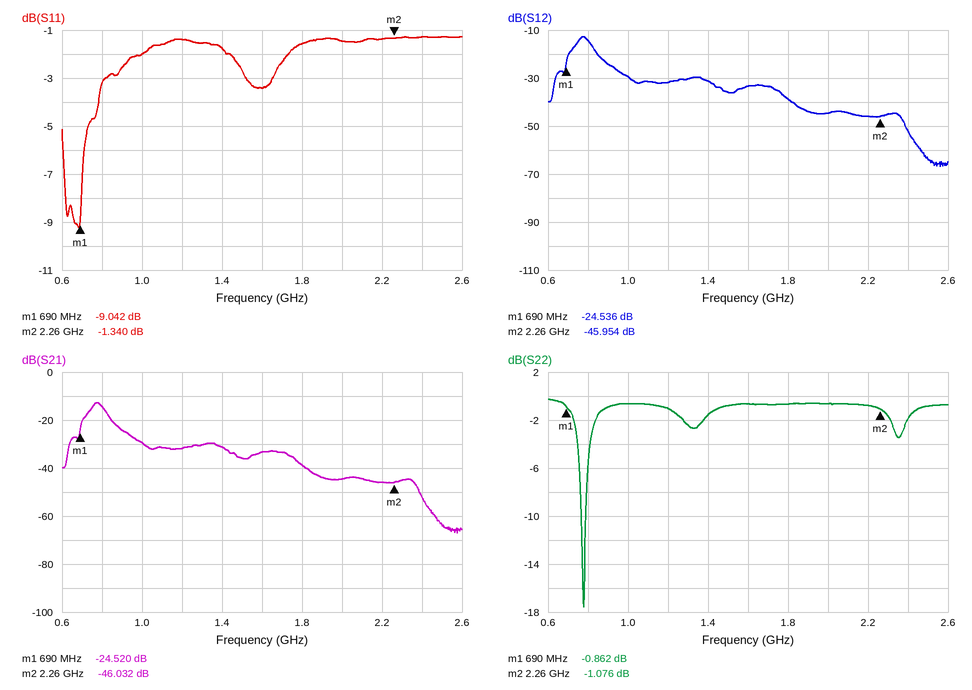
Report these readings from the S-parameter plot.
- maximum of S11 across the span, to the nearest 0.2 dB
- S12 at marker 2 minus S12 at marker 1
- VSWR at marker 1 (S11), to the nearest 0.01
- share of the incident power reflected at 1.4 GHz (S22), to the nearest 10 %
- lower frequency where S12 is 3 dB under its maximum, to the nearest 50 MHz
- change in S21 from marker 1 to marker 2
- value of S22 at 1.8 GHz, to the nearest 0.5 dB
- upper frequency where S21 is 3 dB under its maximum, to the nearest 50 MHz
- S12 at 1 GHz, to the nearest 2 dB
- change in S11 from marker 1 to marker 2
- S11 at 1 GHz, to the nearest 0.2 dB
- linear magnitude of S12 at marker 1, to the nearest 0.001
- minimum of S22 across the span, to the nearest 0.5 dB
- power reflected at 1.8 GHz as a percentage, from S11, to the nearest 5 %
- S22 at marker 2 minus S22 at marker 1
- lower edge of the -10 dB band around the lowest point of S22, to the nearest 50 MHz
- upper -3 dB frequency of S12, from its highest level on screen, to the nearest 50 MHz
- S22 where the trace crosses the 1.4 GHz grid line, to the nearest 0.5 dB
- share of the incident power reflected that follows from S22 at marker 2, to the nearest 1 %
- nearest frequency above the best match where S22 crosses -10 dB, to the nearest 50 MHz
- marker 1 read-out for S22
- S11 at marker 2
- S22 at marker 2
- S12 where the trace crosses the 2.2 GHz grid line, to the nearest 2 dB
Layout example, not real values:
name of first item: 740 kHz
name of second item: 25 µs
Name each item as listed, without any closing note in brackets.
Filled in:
maximum of S11 across the span, to the nearest 0.2 dB: -1.2 dB
S12 at marker 2 minus S12 at marker 1: -21.418 dB
VSWR at marker 1 (S11), to the nearest 0.01: 2.09
share of the incident power reflected at 1.4 GHz (S22), to the nearest 10 %: 70 %
lower frequency where S12 is 3 dB under its maximum, to the nearest 50 MHz: 750 MHz
change in S21 from marker 1 to marker 2: -21.512 dB
value of S22 at 1.8 GHz, to the nearest 0.5 dB: -0.5 dB
upper frequency where S21 is 3 dB under its maximum, to the nearest 50 MHz: 800 MHz
S12 at 1 GHz, to the nearest 2 dB: -30 dB
change in S11 from marker 1 to marker 2: 7.702 dB
S11 at 1 GHz, to the nearest 0.2 dB: -2.0 dB
linear magnitude of S12 at marker 1, to the nearest 0.001: 0.059
minimum of S22 across the span, to the nearest 0.5 dB: -17.5 dB
power reflected at 1.8 GHz as a percentage, from S11, to the nearest 5 %: 70 %
S22 at marker 2 minus S22 at marker 1: -0.214 dB
lower edge of the -10 dB band around the lowest point of S22, to the nearest 50 MHz: 750 MHz
upper -3 dB frequency of S12, from its highest level on screen, to the nearest 50 MHz: 800 MHz
S22 where the trace crosses the 1.4 GHz grid line, to the nearest 0.5 dB: -1.5 dB
share of the incident power reflected that follows from S22 at marker 2, to the nearest 1 %: 78 %
nearest frequency above the best match where S22 crosses -10 dB, to the nearest 50 MHz: 800 MHz
marker 1 read-out for S22: -0.862 dB
S11 at marker 2: -1.340 dB
S22 at marker 2: -1.076 dB
S12 where the trace crosses the 2.2 GHz grid line, to the nearest 2 dB: -46 dB
